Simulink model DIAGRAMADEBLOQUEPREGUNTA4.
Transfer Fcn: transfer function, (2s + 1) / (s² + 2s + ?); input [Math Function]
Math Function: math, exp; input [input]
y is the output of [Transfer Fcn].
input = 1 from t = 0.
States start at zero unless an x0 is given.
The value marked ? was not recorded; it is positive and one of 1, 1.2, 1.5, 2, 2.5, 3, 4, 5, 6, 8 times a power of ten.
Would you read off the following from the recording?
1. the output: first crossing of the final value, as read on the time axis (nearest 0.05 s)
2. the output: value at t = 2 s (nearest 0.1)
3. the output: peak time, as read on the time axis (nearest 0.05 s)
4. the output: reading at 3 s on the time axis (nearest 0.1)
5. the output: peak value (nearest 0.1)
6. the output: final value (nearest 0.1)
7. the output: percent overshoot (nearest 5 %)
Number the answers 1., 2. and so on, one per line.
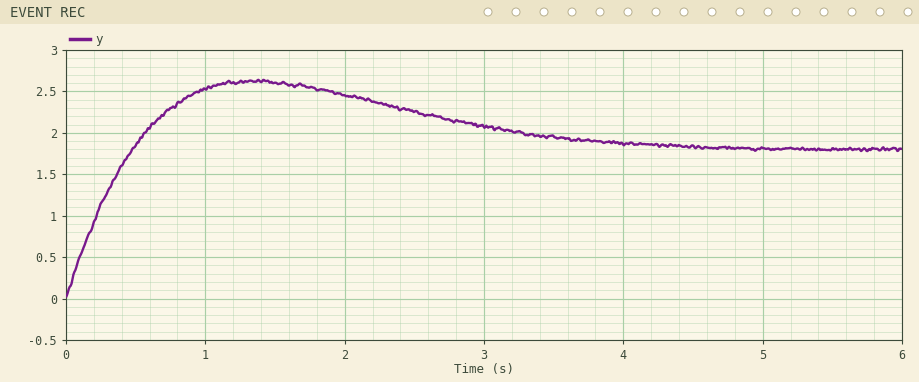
1. 0.50 s
2. 2.5
3. 1.35 s
4. 2.1
5. 2.6
6. 1.8
7. 45 %
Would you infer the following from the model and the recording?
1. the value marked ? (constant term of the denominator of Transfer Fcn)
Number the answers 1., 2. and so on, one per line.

1. 1.5
